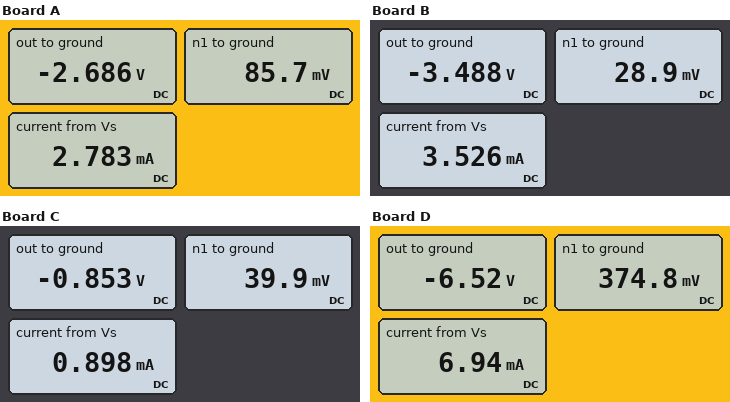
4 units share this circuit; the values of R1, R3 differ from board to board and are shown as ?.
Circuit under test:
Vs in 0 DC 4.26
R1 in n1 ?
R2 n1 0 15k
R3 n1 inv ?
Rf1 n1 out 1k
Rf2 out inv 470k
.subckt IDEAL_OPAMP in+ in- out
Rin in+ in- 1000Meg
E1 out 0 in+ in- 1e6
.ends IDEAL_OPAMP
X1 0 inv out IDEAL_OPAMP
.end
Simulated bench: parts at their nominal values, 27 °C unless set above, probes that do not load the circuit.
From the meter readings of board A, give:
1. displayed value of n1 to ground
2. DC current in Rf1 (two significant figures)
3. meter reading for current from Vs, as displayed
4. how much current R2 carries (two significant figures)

85.7 mV
2.8 mA
2.783 mA
5.7 µA
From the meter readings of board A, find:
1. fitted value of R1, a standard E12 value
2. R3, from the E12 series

1.5 kΩ
15 kΩ
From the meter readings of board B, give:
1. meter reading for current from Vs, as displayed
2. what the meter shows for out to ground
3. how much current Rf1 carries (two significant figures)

3.526 mA
-3.488 V
3.5 mA
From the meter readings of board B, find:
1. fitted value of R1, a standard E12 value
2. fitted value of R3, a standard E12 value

1.2 kΩ
3.9 kΩ
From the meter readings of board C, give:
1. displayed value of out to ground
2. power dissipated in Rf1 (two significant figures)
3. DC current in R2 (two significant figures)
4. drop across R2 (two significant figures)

-0.853 V
800 µW
2.7 µA
40 mV
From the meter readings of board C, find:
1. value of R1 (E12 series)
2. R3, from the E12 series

4.7 kΩ
22 kΩ
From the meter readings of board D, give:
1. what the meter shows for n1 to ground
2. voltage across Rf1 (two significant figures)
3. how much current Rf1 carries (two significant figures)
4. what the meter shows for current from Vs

374.8 mV
6.9 V
6.9 mA
6.94 mA
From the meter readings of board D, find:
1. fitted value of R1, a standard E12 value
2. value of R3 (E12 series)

560 Ω
27 kΩ
